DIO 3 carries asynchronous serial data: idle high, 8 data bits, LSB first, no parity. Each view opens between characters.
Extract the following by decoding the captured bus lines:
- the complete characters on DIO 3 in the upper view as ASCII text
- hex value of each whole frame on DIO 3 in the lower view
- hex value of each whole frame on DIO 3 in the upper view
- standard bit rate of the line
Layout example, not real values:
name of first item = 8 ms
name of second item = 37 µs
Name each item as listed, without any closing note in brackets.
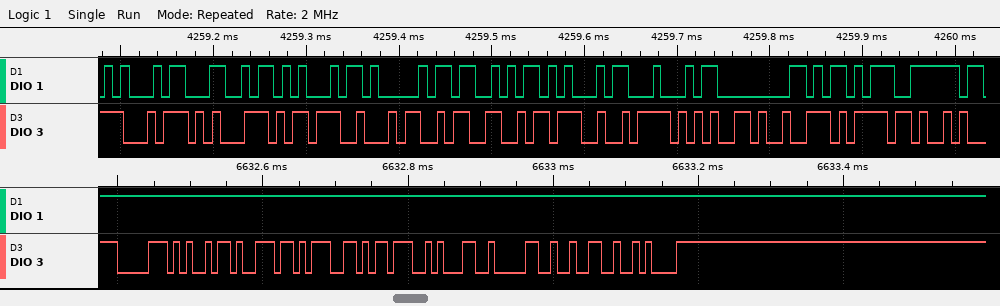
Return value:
the complete characters on DIO 3 in the upper view as ASCII text = "tq;43;zero"
hex value of each whole frame on DIO 3 in the lower view = 70, 69, 6E, 67, 3B, 31, 30, 32, 0A
hex value of each whole frame on DIO 3 in the upper view = 74, 71, 3B, 34, 33, 3B, 7A, 65, 72, 6F
standard bit rate of the line = 115200 baud
